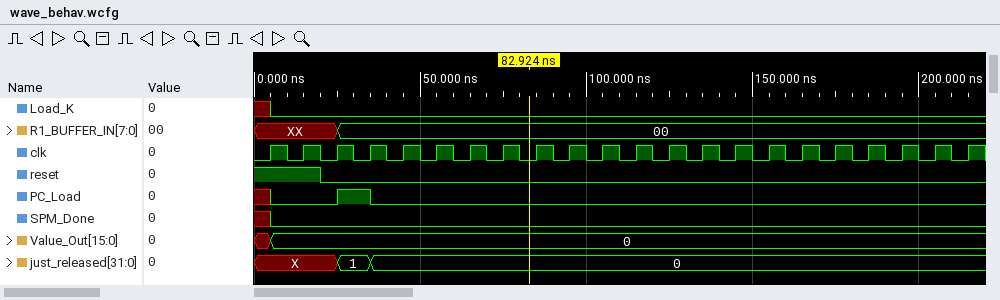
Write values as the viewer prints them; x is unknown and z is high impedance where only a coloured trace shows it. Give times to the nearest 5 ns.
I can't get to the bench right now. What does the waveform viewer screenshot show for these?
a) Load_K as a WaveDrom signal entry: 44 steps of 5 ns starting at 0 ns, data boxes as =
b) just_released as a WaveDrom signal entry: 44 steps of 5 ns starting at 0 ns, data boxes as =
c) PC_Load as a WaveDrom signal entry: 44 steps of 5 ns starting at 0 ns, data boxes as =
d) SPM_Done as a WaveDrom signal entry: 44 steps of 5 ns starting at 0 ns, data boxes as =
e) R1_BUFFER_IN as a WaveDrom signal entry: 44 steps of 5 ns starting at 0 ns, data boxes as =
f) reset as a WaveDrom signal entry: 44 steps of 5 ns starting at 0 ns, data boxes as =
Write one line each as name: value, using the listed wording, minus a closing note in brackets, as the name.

Load_K as a WaveDrom signal entry: 44 steps of 5 ns starting at 0 ns, data boxes as =: {name: 'Load_K', wave: 'x0..........................................'}
just_released as a WaveDrom signal entry: 44 steps of 5 ns starting at 0 ns, data boxes as =: {name: 'just_released', wave: 'x....=.=....................................', data: '1 0'}
PC_Load as a WaveDrom signal entry: 44 steps of 5 ns starting at 0 ns, data boxes as =: {name: 'PC_Load', wave: 'x0...1.0....................................'}
SPM_Done as a WaveDrom signal entry: 44 steps of 5 ns starting at 0 ns, data boxes as =: {name: 'SPM_Done', wave: 'x0..........................................'}
R1_BUFFER_IN as a WaveDrom signal entry: 44 steps of 5 ns starting at 0 ns, data boxes as =: {name: 'R1_BUFFER_IN', wave: 'x....=......................................', data: '00'}
reset as a WaveDrom signal entry: 44 steps of 5 ns starting at 0 ns, data boxes as =: {name: 'reset', wave: '1...0.......................................'}
